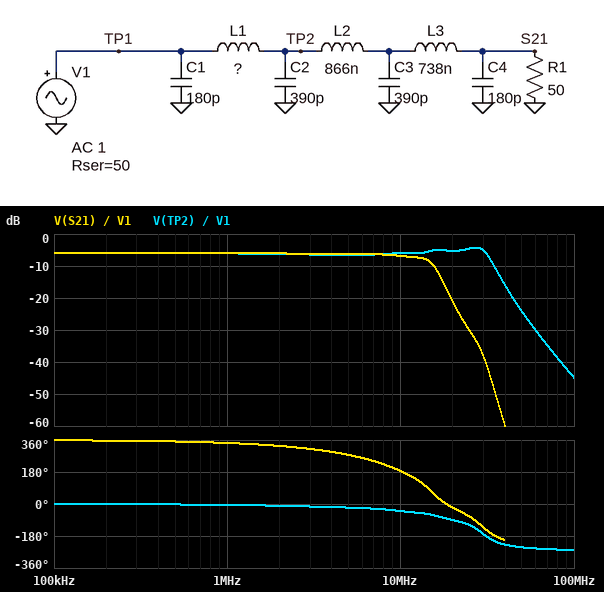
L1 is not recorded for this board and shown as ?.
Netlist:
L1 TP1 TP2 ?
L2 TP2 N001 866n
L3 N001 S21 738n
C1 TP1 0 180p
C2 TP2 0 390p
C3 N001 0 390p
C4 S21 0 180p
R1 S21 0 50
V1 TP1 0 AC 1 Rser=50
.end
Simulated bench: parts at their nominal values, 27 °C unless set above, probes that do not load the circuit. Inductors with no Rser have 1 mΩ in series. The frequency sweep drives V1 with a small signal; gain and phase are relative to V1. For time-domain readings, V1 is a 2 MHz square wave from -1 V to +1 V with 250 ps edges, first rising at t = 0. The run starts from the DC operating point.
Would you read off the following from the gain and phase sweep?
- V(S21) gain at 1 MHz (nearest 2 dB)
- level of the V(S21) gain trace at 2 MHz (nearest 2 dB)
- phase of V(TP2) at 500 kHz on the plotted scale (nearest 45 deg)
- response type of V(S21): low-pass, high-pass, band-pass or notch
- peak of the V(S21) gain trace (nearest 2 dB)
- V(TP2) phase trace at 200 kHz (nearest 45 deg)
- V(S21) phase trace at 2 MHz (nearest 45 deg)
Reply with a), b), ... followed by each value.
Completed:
a) -6 dB
b) -6 dB
c) 0 deg
d) low-pass
e) -6 dB
f) 0 deg
g) 315 deg
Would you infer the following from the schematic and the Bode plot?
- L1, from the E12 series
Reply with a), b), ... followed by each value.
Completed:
a) 220 nH
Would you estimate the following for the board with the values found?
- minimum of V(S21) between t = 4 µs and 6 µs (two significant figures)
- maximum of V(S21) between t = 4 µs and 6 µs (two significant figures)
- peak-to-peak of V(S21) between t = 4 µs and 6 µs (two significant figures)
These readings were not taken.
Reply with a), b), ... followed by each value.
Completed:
a) -610 mV
b) 610 mV
c) 1.2 V
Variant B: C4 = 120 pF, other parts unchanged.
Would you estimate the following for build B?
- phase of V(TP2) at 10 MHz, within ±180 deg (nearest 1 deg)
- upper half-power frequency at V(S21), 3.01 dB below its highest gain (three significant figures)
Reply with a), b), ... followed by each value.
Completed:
a) -39 deg
b) 14.5 MHz
